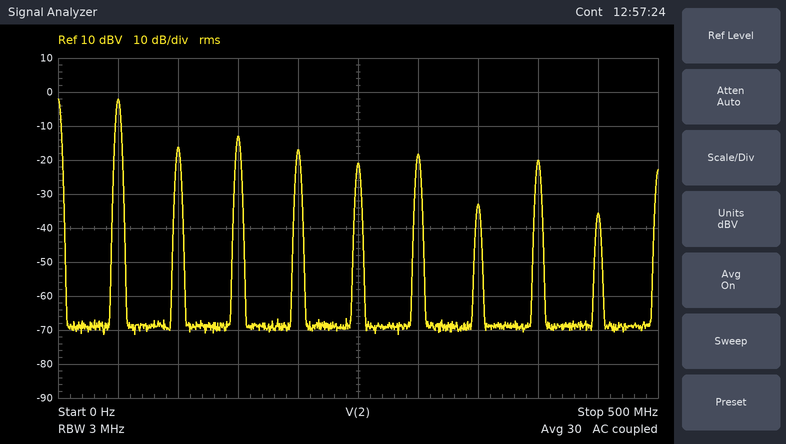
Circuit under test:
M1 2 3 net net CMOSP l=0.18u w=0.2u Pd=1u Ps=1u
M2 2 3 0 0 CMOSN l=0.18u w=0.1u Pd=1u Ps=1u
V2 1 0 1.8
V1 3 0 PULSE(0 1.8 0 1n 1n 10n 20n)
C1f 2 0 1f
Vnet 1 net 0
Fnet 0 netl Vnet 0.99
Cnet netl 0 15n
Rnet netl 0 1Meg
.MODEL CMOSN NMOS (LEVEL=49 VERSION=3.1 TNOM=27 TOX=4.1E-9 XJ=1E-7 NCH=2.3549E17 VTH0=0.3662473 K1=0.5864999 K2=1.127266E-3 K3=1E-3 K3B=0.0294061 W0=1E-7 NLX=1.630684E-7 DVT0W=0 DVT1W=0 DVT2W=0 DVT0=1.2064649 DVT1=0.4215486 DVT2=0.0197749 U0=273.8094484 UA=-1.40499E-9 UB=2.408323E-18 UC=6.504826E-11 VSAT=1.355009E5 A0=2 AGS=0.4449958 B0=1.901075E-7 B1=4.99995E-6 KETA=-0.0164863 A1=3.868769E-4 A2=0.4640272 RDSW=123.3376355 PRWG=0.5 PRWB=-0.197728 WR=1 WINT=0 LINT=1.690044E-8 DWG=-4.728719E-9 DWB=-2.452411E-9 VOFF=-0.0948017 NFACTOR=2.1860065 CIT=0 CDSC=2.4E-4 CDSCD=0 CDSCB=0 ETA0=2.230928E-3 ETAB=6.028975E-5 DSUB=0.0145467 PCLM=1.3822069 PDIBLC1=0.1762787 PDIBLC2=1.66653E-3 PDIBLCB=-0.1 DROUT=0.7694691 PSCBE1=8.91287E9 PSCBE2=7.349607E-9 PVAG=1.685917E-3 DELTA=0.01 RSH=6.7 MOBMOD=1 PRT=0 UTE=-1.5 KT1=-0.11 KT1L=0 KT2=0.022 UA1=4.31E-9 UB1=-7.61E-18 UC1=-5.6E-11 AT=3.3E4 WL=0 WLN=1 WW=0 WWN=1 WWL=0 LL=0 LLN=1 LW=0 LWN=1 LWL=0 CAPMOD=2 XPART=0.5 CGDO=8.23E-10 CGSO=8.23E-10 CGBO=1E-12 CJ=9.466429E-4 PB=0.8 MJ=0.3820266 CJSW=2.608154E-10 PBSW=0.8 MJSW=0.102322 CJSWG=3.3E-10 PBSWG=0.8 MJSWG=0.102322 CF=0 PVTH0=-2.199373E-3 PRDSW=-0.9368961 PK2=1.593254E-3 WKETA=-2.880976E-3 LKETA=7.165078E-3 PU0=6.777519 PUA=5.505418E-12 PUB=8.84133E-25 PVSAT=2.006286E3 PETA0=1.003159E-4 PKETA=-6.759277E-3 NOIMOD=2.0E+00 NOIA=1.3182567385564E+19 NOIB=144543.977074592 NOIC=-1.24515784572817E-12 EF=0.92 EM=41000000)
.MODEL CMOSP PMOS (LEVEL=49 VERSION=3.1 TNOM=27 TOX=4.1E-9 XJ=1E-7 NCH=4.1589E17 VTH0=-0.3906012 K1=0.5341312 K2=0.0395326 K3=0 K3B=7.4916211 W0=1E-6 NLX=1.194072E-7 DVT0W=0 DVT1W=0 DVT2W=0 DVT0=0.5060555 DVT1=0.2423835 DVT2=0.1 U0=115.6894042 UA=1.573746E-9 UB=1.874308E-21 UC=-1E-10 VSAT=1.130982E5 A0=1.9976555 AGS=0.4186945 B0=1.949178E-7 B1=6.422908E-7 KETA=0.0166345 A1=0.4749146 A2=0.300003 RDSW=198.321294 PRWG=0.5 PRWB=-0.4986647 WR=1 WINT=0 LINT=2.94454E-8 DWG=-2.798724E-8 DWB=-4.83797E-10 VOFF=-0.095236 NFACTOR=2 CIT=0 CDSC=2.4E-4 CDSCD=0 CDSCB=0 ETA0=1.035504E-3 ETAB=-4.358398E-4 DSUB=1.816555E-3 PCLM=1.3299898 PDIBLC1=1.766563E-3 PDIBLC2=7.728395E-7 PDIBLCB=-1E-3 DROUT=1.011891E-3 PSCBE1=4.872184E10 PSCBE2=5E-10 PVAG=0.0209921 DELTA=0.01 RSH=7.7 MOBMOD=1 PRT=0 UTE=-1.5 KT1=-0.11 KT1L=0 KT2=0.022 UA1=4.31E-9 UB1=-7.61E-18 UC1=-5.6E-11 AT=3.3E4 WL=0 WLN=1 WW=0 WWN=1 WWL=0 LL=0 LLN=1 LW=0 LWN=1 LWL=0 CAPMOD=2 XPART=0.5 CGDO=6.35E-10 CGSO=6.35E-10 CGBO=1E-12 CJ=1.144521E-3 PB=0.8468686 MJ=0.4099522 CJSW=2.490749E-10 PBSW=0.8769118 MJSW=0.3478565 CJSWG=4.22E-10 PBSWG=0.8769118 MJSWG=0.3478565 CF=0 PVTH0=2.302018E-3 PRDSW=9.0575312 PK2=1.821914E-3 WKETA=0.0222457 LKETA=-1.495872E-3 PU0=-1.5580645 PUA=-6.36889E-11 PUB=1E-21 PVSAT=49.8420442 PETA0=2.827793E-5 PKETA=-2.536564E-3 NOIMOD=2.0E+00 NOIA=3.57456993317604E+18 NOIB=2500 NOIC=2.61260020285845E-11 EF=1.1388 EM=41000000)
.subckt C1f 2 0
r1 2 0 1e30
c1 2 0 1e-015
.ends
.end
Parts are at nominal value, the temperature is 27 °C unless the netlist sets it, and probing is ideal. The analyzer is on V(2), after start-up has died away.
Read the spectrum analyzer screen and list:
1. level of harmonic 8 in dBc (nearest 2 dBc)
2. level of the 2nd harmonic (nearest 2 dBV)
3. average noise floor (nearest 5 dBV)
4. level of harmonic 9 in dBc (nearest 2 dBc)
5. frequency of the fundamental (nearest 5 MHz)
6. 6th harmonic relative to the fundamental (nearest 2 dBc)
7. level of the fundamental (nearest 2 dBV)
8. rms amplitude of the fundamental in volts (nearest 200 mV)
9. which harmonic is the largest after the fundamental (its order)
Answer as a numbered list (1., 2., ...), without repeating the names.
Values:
1. -18 dBc
2. -16 dBV
3. -70 dBV
4. -34 dBc
5. 50 MHz
6. -16 dBc
7. -2 dBV
8. 800 mV
9. 3
